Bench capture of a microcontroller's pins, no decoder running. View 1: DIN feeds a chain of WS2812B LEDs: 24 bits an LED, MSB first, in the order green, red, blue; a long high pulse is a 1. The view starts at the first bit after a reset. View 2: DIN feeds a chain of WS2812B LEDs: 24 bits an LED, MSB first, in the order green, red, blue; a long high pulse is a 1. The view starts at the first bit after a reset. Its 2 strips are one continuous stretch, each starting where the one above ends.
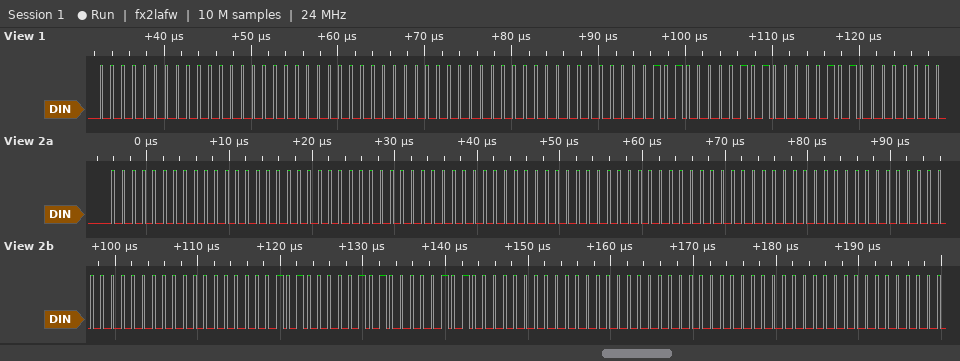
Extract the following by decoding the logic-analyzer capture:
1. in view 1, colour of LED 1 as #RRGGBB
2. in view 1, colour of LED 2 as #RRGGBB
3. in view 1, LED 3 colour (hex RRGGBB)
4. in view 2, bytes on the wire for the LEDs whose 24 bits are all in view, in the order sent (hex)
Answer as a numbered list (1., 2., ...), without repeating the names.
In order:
1. #000000
2. #000000
3. #141414
4. 00 00 00 00 00 00 00 00 00 00 00 00 14 14 14 00 00 00
